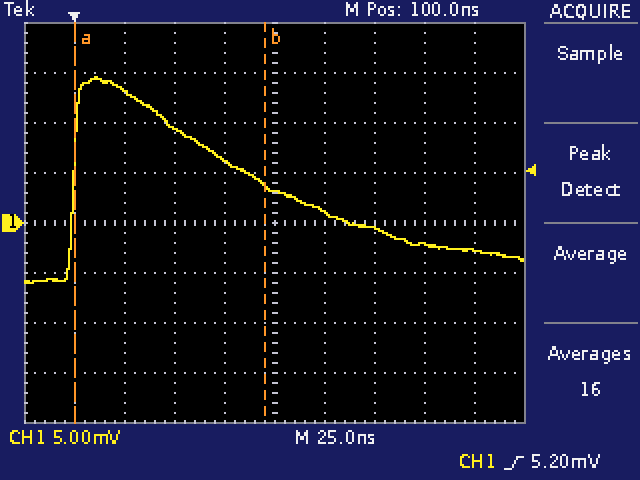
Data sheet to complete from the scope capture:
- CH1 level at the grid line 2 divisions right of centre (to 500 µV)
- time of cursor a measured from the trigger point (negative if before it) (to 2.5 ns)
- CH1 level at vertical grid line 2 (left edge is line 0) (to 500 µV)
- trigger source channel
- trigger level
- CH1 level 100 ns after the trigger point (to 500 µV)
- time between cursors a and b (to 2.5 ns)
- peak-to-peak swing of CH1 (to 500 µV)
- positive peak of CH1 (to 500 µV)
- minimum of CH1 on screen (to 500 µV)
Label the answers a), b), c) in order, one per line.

a) -500 µV
b) 0.0 ns
c) 13.0 mV
d) CH1
e) 5.20 mV
f) 3.0 mV
g) 95.0 ns
h) 20.5 mV
i) 14.5 mV
j) -6.0 mV
